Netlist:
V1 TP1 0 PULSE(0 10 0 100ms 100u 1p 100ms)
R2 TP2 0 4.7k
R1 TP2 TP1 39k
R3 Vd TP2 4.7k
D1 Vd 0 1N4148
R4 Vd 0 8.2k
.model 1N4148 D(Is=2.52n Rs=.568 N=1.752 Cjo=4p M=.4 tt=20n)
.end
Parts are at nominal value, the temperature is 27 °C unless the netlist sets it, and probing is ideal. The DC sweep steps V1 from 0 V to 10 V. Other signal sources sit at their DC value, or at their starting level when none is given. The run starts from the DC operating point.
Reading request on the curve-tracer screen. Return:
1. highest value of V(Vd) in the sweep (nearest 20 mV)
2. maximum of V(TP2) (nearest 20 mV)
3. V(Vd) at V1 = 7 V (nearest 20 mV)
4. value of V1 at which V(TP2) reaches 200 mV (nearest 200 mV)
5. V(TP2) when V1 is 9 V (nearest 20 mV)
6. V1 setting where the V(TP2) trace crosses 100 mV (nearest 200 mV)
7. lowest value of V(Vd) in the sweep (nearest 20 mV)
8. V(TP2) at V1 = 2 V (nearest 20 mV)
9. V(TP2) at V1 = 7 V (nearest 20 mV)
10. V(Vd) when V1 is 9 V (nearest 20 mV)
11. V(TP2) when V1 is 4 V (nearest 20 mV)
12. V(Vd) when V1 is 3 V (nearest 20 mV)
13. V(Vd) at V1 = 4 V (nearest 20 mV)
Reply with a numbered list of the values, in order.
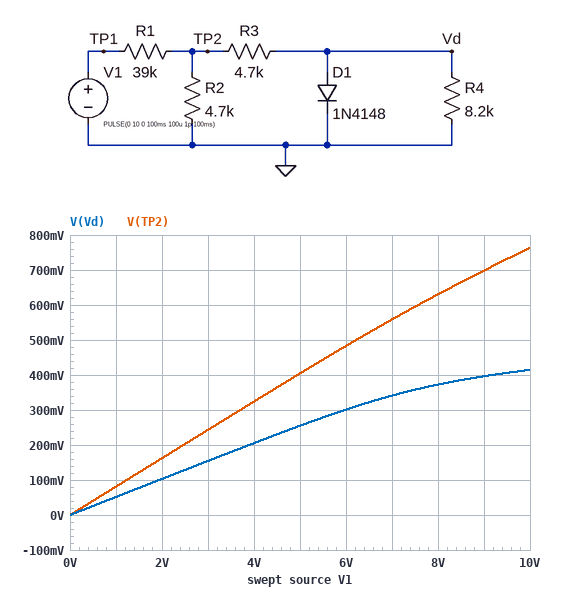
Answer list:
1. 420 mV
2. 760 mV
3. 340 mV
4. 2.4 V
5. 700 mV
6. 1.2 V
7. 0 V
8. 160 mV
9. 560 mV
10. 400 mV
11. 320 mV
12. 160 mV
13. 200 mV
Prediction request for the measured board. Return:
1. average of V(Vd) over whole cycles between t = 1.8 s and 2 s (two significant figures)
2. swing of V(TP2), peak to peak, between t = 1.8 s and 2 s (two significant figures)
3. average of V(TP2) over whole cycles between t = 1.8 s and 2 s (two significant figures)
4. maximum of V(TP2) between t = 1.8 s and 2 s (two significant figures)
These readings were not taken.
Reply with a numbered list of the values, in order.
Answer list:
1. 240 mV
2. 760 mV
3. 400 mV
4. 760 mV
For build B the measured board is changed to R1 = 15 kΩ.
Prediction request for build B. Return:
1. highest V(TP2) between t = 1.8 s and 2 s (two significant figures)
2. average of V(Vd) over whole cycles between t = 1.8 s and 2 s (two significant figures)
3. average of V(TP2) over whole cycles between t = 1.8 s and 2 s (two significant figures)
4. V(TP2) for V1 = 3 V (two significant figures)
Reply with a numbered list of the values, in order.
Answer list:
1. 1.6 V
2. 370 mV
3. 840 mV
4. 550 mV
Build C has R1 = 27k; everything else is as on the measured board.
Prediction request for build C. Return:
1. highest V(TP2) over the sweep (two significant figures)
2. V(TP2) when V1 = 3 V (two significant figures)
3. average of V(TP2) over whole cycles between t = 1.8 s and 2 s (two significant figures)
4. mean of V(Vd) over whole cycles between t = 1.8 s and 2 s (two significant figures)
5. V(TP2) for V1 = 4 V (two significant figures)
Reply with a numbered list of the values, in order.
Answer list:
1. 1.0 V
2. 340 mV
3. 540 mV
4. 300 mV
5. 450 mV
